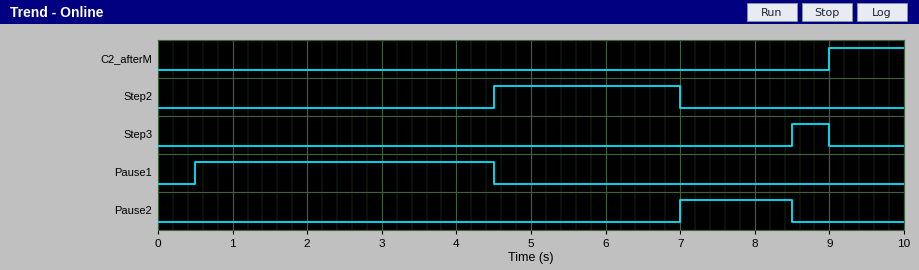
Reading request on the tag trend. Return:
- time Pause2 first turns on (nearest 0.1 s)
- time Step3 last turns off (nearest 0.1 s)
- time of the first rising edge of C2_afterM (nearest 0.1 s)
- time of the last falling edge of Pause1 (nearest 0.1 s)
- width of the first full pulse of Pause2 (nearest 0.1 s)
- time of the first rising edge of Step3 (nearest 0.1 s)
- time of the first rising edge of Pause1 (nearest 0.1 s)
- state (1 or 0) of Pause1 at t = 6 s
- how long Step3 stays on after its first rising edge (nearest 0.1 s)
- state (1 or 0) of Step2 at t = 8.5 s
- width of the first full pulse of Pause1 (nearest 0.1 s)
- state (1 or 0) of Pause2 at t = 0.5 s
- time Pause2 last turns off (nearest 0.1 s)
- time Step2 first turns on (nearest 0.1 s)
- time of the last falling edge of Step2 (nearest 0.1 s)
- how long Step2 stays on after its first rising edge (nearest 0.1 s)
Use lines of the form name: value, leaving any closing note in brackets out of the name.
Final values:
time Pause2 first turns on: 7.0 s
time Step3 last turns off: 9.0 s
time of the first rising edge of C2_afterM: 9.0 s
time of the last falling edge of Pause1: 4.5 s
width of the first full pulse of Pause2: 1.5 s
time of the first rising edge of Step3: 8.5 s
time of the first rising edge of Pause1: 0.5 s
state (1 or 0) of Pause1 at t = 6 s: 0
how long Step3 stays on after its first rising edge: 0.5 s
state (1 or 0) of Step2 at t = 8.5 s: 0
width of the first full pulse of Pause1: 4.0 s
state (1 or 0) of Pause2 at t = 0.5 s: 0
time Pause2 last turns off: 8.5 s
time Step2 first turns on: 4.5 s
time of the last falling edge of Step2: 7.0 s
how long Step2 stays on after its first rising edge: 2.5 s
